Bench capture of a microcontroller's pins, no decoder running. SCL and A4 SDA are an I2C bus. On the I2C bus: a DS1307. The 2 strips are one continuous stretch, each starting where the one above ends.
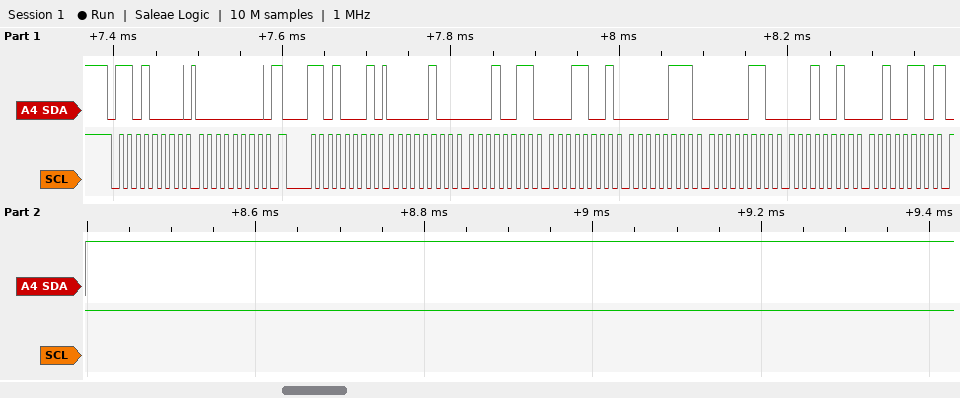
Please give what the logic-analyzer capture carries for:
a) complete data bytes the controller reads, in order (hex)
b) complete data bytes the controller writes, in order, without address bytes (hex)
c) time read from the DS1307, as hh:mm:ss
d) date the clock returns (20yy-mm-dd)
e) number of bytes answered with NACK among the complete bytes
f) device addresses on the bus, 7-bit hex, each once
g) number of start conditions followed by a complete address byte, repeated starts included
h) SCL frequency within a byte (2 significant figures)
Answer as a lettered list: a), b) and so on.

a) 04 13 19 07 06 12 26
b) 00
c) 19:13:04
d) 2026-12-06
e) 1
f) 0x68
g) 2
h) 100 kHz
